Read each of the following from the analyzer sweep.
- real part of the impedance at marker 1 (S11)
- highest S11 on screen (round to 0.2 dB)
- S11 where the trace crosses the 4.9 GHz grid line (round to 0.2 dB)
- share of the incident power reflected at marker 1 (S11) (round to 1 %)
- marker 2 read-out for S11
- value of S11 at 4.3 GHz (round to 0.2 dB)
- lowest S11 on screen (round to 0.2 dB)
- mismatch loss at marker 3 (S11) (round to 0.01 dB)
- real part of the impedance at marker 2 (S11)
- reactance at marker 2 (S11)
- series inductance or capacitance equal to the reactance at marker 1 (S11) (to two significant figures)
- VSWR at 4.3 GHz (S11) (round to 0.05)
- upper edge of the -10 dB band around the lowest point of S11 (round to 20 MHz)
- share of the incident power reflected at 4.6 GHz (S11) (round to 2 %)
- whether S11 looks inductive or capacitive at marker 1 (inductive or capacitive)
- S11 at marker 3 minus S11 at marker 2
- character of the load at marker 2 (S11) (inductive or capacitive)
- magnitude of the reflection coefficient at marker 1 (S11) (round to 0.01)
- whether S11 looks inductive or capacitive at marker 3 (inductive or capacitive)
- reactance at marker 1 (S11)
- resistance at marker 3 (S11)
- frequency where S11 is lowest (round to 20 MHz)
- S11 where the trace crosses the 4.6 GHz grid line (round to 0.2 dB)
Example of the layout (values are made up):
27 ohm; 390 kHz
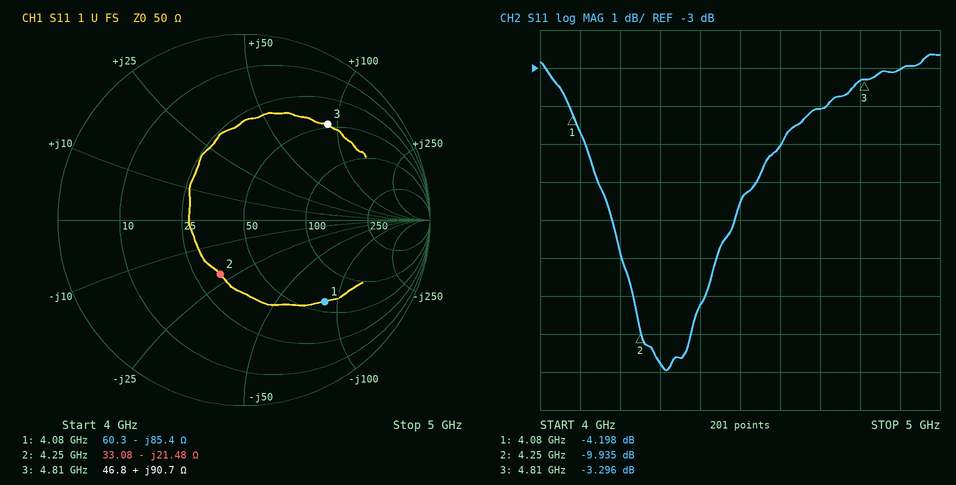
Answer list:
60.3 Ω; -2.6 dB; -3.0 dB; 38 %; -9.935 dB; -10.8 dB; -11.0 dB; 2.74 dB; 33.08 Ω; -21.48 Ω; 460 fF; 1.80; 4.38 GHz; 32 %; capacitive; 6.639 dB; capacitive; 0.62; inductive; -85.4 Ω; 46.8 Ω; 4.32 GHz; -5.0 dB
